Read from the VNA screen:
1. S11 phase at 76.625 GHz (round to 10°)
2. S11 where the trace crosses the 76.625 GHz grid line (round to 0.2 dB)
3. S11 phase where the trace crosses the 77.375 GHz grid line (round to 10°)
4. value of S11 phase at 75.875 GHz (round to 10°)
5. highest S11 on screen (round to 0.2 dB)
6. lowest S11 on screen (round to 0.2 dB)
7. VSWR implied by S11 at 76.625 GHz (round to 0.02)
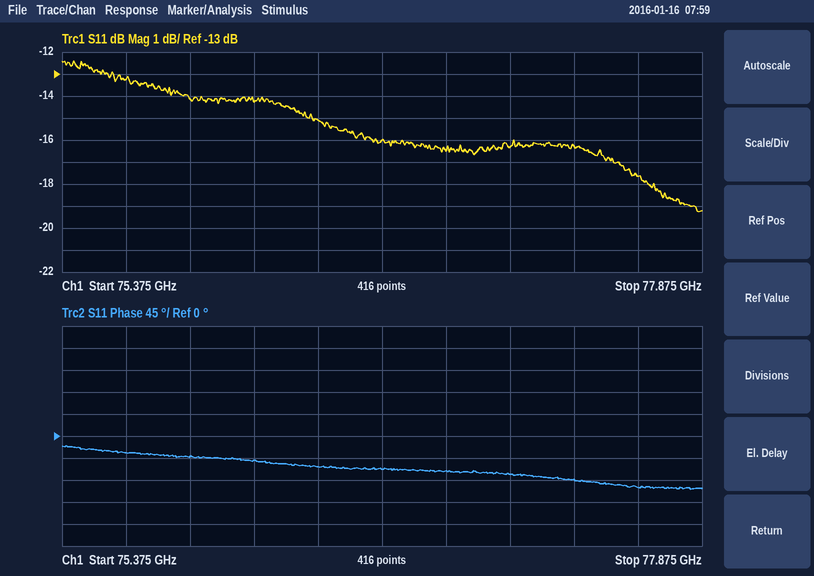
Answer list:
-70°
-16.0 dB
-90°
-40°
-12.4 dB
-19.2 dB
1.38
